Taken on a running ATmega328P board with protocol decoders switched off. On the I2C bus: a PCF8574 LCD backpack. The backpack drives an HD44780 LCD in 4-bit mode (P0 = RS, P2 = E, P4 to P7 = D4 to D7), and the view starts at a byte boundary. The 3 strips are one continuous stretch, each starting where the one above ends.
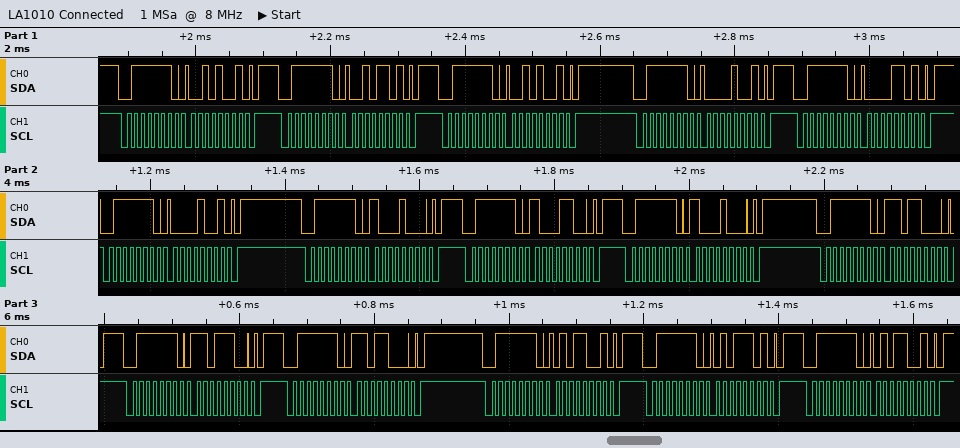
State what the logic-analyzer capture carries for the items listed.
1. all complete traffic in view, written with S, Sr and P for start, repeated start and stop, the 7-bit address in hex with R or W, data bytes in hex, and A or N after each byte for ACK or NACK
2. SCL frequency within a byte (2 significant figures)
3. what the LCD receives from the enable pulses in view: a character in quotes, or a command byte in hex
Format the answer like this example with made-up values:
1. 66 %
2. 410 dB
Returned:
1. S 3FW A 29 A P S 3FW A 2D A P S 3FW A 29 A P S 3FW A 09 A P S 3FW A 0D A P S 3FW A 09 A P S 3FW A 88 A P S 3FW A 8C A P S 3FW A 88 A P S 3FW A D8 A P S 3FW A DC A P S 3FW A D8 A P S 3FW A 59 A P S 3FW A 5D A P S 3FW A 59 A P
2. 100 kHz
3. ' ' 0x8D
